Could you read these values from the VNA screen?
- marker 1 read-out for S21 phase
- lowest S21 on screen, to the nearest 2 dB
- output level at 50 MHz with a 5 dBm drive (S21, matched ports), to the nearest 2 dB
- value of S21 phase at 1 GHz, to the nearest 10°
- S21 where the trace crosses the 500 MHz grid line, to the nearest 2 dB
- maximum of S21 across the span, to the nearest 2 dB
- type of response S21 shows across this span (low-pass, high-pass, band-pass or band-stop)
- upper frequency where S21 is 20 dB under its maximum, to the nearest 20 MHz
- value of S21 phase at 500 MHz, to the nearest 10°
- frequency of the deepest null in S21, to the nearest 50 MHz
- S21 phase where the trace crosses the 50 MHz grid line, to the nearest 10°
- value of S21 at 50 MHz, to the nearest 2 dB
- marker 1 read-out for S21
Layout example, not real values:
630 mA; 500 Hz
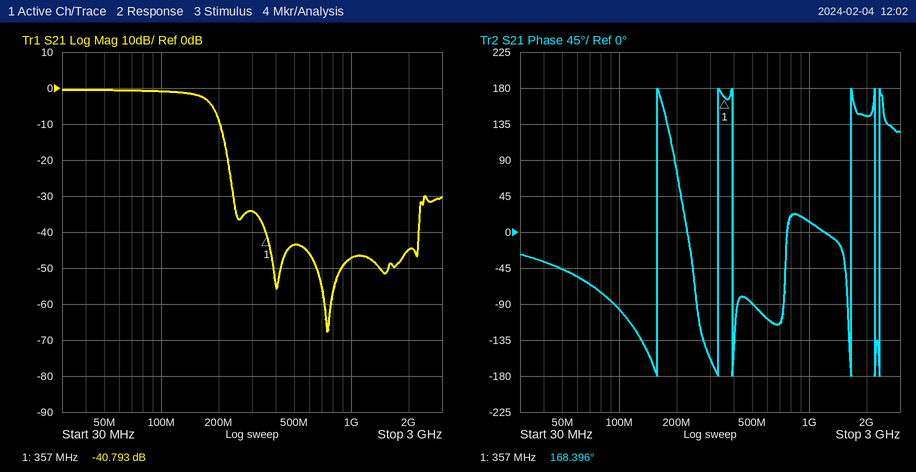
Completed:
168.396°; -68 dB; 4 dBm; 10°; -44 dB; 0 dB; low-pass; 220 MHz; -90°; 750 MHz; -50°; 0 dB; -40.793 dB
